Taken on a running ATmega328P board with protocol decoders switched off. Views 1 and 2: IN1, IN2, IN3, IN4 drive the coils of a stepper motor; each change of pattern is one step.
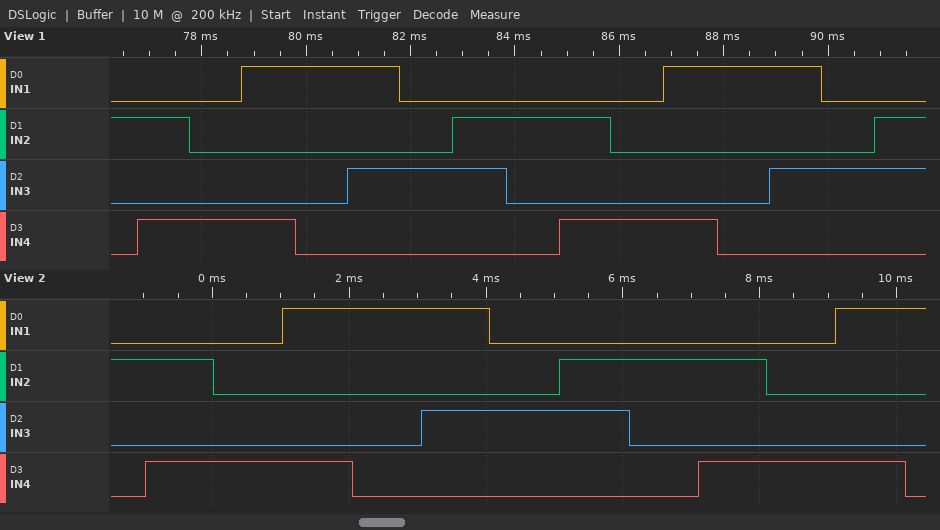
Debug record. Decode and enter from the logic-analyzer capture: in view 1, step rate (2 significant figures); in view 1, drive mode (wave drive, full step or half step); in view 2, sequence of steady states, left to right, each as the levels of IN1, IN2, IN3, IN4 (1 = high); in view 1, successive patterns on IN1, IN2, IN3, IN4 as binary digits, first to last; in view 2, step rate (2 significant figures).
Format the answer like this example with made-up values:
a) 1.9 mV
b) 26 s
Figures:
a) 990 steps/s
b) half step
c) 0100 0101 0001 1001 1000 1010 0010 0110 0100 0101 0001 1001 1000
d) 0100 0101 0001 1001 1000 1010 0010 0110 0100 0101 0001 1001 1000 1010 0010 0110
e) 990 steps/s
